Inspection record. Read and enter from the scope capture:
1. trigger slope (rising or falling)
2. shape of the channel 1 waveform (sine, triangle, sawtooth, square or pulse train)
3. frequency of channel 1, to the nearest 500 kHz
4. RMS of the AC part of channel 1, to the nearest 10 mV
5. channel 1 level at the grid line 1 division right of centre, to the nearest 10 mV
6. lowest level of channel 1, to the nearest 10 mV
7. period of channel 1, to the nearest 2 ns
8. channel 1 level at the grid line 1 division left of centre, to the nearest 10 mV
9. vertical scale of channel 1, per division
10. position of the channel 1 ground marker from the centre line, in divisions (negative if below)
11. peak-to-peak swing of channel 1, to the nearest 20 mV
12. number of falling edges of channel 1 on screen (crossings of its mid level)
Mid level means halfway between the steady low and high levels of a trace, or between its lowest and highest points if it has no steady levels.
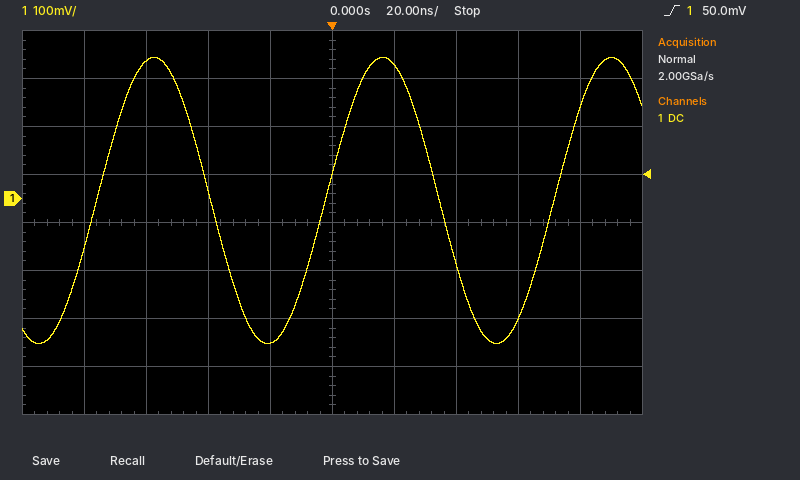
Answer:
rising
sine
13.5 MHz
210 mV
280 mV
-300 mV
74 ns
-300 mV
100 mV
+0.5 div
600 mV
2
